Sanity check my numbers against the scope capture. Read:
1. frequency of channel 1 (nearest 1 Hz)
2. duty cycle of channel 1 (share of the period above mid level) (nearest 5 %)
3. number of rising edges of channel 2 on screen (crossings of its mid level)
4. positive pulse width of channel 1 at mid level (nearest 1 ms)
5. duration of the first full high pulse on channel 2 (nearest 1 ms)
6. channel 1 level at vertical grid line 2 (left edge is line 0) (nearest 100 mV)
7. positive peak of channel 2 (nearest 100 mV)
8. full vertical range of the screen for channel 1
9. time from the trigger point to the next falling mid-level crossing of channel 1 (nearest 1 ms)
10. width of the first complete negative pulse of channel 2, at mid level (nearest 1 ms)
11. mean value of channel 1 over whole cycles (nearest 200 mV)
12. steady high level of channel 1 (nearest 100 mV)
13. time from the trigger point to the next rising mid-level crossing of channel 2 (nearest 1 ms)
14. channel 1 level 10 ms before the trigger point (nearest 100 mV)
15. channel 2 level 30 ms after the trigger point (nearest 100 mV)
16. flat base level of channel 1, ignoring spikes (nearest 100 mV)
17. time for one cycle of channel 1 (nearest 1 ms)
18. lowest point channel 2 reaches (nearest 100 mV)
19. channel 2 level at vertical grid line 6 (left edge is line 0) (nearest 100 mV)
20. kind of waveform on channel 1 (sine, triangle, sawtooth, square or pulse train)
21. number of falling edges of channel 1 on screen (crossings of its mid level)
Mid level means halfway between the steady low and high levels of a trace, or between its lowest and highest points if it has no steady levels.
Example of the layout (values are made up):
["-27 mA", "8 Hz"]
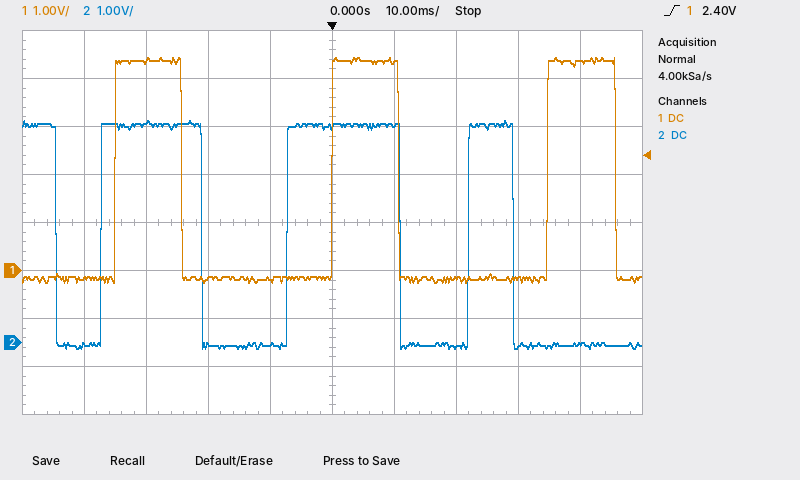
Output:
["29 Hz", "30 %", "3", "11 ms", "16 ms", "4.4 V", "4.6 V", "8 V", "11 ms", "7 ms", "1.2 V", "4.4 V", "22 ms", "-200 mV", "-100 mV", "-200 mV", "35 ms", "-100 mV", "4.5 V", "pulse train", "3"]
